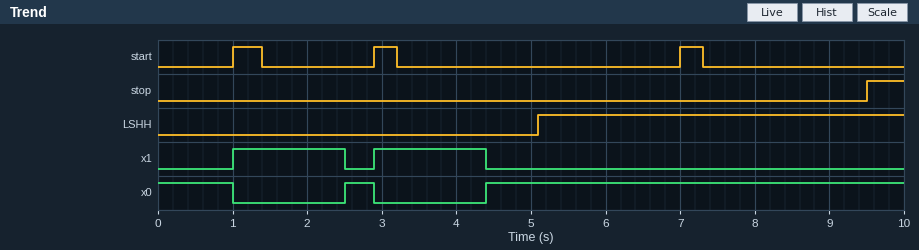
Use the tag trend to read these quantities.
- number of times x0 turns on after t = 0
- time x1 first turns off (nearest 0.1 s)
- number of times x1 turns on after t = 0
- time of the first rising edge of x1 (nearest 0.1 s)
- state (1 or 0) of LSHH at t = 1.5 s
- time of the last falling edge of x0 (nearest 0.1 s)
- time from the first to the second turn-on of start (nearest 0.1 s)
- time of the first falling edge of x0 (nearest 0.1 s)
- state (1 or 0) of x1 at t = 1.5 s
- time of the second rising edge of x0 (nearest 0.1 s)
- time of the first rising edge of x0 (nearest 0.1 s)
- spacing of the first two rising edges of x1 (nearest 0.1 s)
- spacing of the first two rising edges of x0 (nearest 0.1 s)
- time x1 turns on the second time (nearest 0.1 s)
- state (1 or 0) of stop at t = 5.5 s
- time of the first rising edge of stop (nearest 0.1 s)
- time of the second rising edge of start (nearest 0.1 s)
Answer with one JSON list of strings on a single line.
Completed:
["2", "2.5 s", "2", "1.0 s", "0", "2.9 s", "1.9 s", "1.0 s", "1", "4.4 s", "2.5 s", "1.9 s", "1.9 s", "2.9 s", "0", "9.5 s", "2.9 s"]
